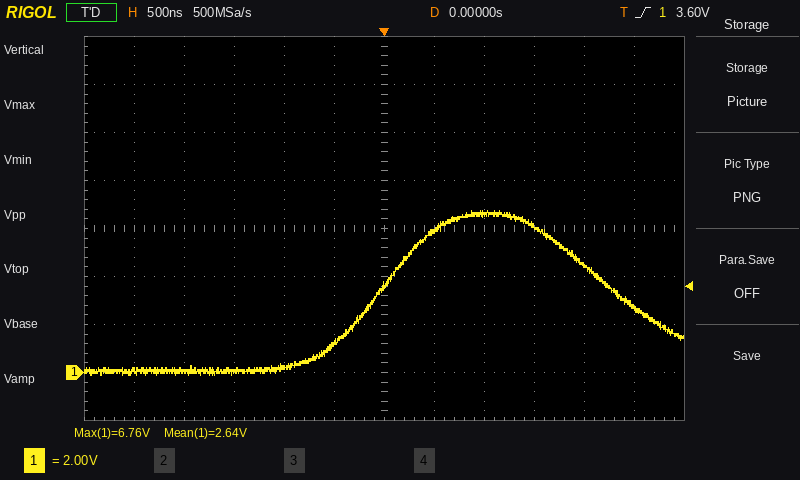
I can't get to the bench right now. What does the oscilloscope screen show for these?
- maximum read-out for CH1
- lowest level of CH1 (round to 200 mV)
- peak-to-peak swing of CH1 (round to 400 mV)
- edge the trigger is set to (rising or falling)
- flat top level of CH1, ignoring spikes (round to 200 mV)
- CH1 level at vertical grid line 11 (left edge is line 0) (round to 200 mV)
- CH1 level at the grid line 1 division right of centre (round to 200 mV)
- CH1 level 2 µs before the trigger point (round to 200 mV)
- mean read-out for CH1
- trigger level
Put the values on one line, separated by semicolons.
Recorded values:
6.76 V; -200 mV; 6.8 V; rising; 6.6 V; 2.6 V; 5.8 V; 0.0 V; 2.64 V; 3.60 V
